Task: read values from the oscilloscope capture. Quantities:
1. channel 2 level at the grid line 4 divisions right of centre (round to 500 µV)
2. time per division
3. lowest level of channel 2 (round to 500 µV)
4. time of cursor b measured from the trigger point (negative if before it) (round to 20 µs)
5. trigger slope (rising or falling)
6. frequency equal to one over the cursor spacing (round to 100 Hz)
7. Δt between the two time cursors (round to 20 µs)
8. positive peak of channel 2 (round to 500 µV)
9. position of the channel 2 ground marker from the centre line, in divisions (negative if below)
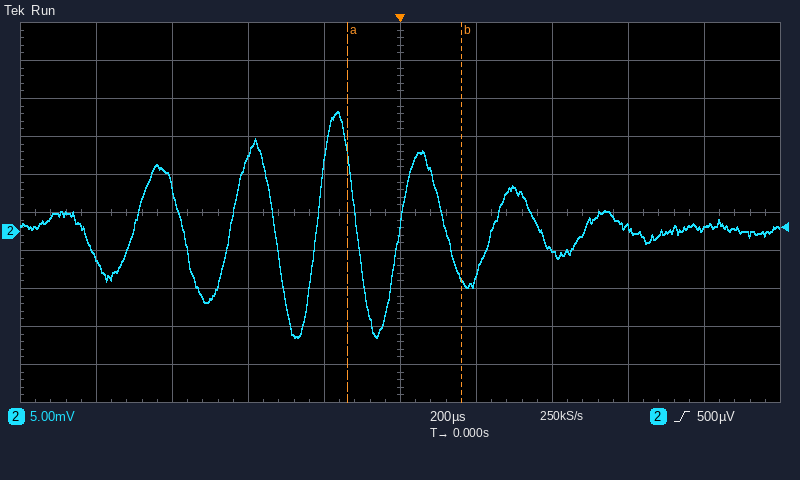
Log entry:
500 µV
200 µs
-14.0 mV
+160 µs
rising
3.3 kHz
300 µs
16.0 mV
-0.5 div
